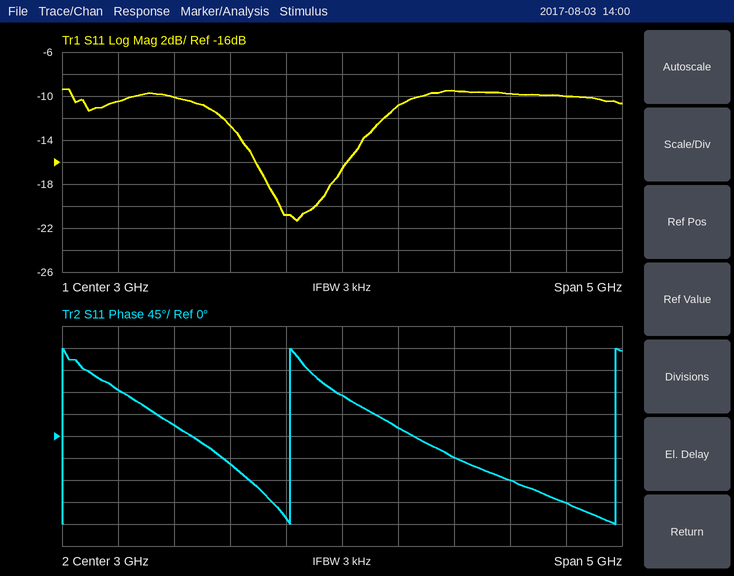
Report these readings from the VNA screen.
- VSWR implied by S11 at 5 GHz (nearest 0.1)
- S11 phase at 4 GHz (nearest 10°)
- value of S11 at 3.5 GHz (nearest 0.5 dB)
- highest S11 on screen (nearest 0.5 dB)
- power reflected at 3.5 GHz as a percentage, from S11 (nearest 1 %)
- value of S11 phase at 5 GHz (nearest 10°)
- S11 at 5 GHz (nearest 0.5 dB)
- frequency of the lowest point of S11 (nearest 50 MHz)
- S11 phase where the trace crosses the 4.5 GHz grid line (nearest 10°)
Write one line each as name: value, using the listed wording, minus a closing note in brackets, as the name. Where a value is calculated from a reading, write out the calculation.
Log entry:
VSWR implied by S11 at 5 GHz: |Γ| = 10^(-10/20) = 0.3162; VSWR = (1 + 0.3162)/(1 − 0.3162) ≈ 1.9
S11 phase at 4 GHz: -40°
value of S11 at 3.5 GHz: -11.0 dB
highest S11 on screen: -9.5 dB
power reflected at 3.5 GHz as a percentage, from S11: 10^(-11/10) ≈ 8 %
value of S11 phase at 5 GHz: -140°
S11 at 5 GHz: -10.0 dB
frequency of the lowest point of S11: 2.60 GHz
S11 phase where the trace crosses the 4.5 GHz grid line: -90°
